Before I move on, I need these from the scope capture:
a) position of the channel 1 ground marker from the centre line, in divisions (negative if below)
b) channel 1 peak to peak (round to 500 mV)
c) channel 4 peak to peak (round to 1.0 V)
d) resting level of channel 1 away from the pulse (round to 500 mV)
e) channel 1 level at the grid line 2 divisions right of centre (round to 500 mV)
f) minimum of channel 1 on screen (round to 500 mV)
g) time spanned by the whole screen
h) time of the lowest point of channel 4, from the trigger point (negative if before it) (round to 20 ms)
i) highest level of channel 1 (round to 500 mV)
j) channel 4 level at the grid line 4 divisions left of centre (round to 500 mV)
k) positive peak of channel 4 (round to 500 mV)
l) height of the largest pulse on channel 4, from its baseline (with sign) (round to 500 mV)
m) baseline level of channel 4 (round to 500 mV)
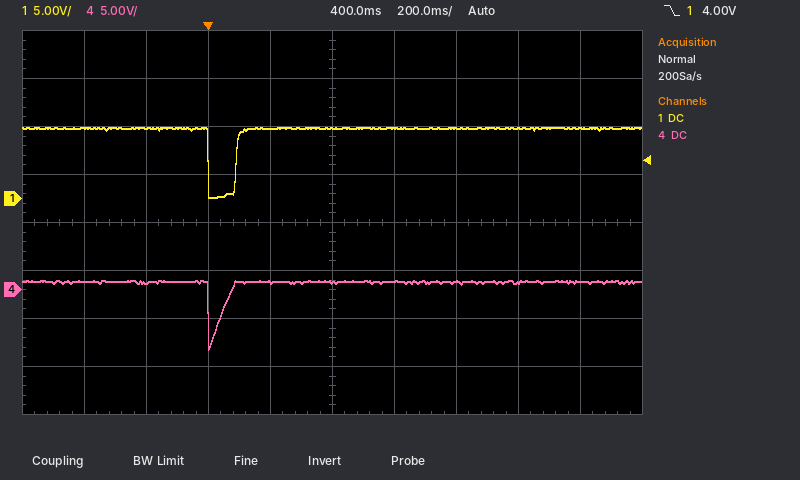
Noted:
+0.5 div
7.5 V
7.0 V
7.5 V
7.5 V
0.0 V
2 s
0 ms
7.5 V
1.0 V
1.0 V
-7.0 V
1.0 V
